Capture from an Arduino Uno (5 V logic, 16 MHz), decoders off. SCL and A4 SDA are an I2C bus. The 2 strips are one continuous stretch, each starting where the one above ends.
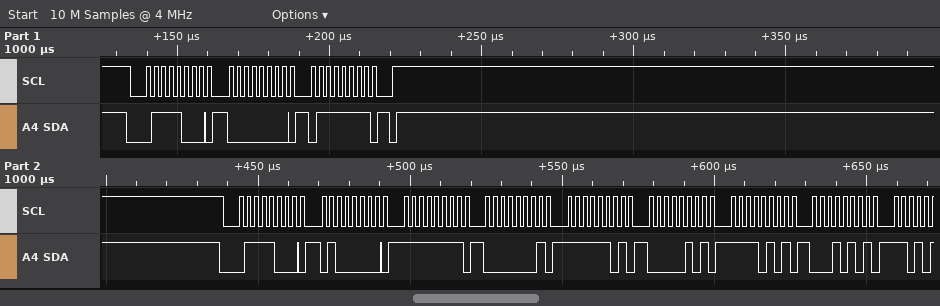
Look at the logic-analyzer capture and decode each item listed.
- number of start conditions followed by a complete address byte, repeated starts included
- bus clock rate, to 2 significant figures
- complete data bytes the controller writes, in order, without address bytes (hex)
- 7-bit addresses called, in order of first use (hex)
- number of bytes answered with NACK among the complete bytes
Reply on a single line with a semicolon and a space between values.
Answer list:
2; 400 kHz; 00 7F 40 FF 01 FD 05 F5 15; 0x3C; 0
